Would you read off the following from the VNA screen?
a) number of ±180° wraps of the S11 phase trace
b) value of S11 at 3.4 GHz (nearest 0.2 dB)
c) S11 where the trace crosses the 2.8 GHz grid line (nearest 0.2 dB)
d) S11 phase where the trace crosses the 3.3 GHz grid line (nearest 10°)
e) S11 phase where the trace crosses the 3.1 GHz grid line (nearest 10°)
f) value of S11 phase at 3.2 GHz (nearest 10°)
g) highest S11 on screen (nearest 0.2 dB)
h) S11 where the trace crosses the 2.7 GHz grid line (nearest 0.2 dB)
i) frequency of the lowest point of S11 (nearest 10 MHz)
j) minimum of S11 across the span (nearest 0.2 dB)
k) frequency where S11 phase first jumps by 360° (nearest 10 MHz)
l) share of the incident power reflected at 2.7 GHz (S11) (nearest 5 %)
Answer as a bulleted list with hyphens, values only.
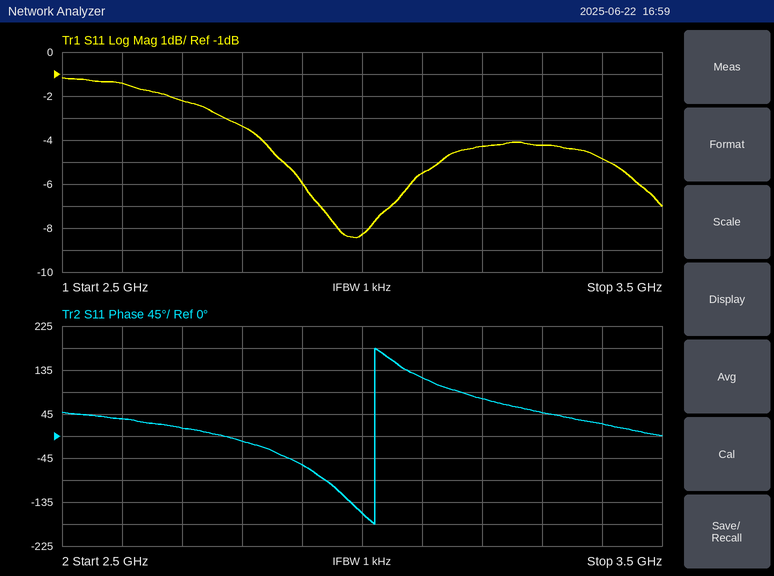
- 1
- -4.8 dB
- -3.4 dB
- 50°
- 120°
- 80°
- -1.2 dB
- -2.2 dB
- 2.99 GHz
- -8.4 dB
- 3.02 GHz
- 60 %
